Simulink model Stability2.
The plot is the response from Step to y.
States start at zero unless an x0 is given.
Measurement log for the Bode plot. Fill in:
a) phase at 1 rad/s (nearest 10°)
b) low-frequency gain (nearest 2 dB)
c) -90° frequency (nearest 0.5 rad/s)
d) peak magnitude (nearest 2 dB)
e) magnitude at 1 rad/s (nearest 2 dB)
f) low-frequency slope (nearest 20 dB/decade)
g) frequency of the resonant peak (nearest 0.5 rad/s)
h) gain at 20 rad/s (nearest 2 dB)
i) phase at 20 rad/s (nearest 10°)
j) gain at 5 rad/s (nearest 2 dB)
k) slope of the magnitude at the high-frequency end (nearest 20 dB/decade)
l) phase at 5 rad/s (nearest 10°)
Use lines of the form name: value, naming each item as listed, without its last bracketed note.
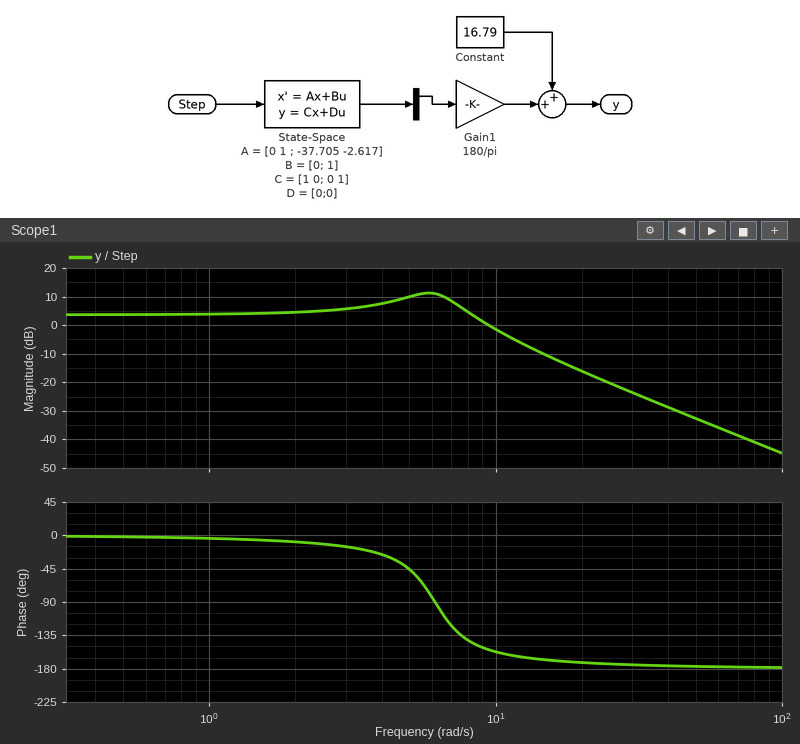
phase at 1 rad/s: 0°
low-frequency gain: 4 dB
-90° frequency: 6.0 rad/s
peak magnitude: 12 dB
magnitude at 1 rad/s: 4 dB
low-frequency slope: 0 dB/decade
frequency of the resonant peak: 6.0 rad/s
gain at 20 rad/s: -16 dB
phase at 20 rad/s: -170°
gain at 5 rad/s: 10 dB
slope of the magnitude at the high-frequency end: -40 dB/decade
phase at 5 rad/s: -50°
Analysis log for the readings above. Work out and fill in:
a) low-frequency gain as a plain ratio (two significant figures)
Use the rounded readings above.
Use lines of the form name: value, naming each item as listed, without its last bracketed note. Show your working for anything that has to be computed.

low-frequency gain as a plain ratio: 10^(4 / 20) = 1.6
